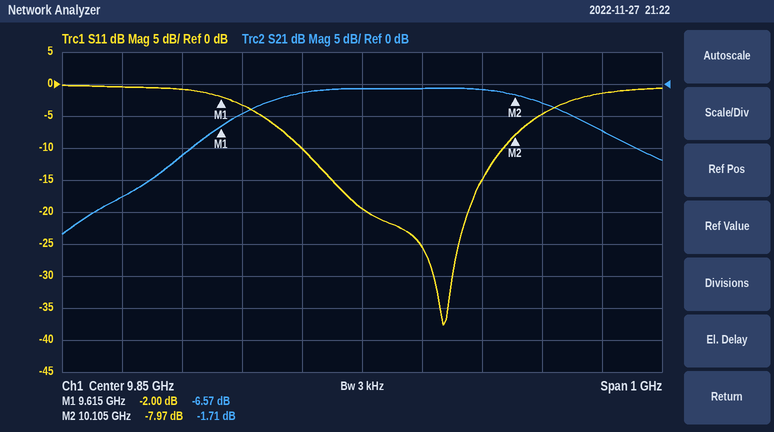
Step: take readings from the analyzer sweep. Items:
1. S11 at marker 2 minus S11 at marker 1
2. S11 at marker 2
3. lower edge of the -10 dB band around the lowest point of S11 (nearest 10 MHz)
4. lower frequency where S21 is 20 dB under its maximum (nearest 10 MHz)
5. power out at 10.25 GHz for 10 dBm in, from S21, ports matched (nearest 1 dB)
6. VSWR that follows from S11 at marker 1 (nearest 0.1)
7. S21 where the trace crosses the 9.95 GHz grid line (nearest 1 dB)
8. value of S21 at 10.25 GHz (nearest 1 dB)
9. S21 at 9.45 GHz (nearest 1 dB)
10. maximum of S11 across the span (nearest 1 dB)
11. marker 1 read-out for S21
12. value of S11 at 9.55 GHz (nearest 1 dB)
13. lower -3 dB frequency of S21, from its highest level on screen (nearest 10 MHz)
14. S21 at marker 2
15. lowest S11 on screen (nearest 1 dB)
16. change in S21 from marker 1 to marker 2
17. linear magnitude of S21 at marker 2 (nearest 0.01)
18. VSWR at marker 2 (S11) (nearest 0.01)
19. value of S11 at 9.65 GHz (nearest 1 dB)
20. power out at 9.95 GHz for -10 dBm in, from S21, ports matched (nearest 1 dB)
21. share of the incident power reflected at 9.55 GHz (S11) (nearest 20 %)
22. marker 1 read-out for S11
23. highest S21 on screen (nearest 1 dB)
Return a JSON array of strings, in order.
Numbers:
["-5.97 dB", "-7.97 dB", "9.75 GHz", "9.39 GHz", "3 dBm", "8.7", "-1 dB", "-7 dB", "-18 dB", "0 dB", "-6.57 dB", "-1 dB", "9.67 GHz", "-1.71 dB", "-38 dB", "4.86 dB", "0.82", "2.33", "-3 dB", "-11 dBm", "80 %", "-2.00 dB", "-1 dB"]
